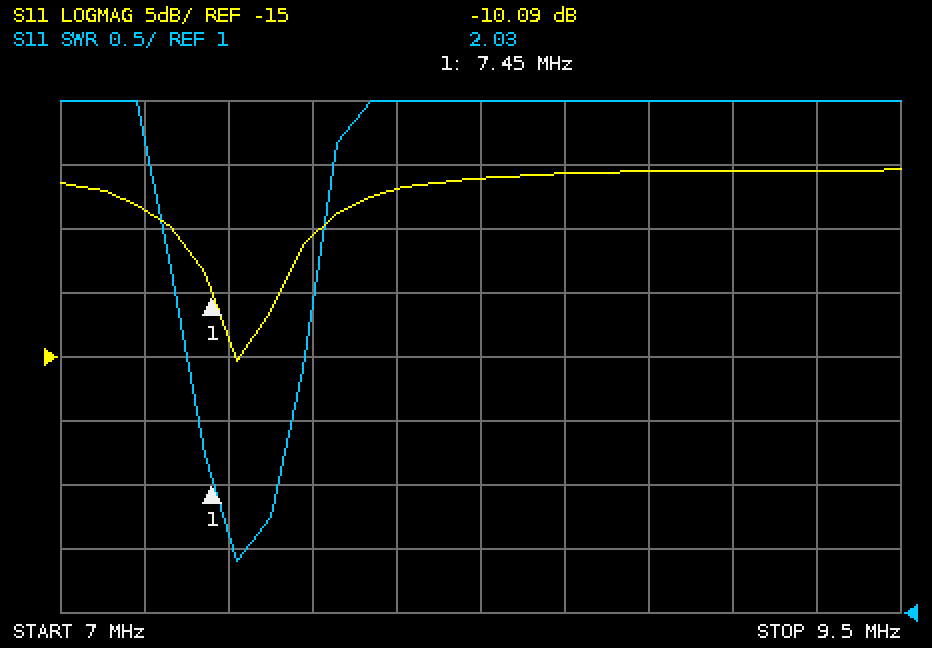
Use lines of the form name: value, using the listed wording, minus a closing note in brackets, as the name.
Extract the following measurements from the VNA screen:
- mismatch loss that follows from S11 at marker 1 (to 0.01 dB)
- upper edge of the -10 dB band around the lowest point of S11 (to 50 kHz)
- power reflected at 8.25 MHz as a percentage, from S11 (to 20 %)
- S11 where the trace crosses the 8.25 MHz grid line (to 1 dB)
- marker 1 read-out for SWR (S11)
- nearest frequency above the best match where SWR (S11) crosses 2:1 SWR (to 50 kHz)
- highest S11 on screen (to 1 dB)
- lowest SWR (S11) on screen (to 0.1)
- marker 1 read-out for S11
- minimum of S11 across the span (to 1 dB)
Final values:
mismatch loss that follows from S11 at marker 1: 0.45 dB
upper edge of the -10 dB band around the lowest point of S11: 7.65 MHz
power reflected at 8.25 MHz as a percentage, from S11: 80 %
S11 where the trace crosses the 8.25 MHz grid line: -1 dB
marker 1 read-out for SWR: 2.03
nearest frequency above the best match where SWR (S11) crosses 2:1 SWR: 7.65 MHz
highest S11 on screen: 0 dB
lowest SWR (S11) on screen: 1.4
marker 1 read-out for S11: -10.09 dB
minimum of S11 across the span: -15 dB
